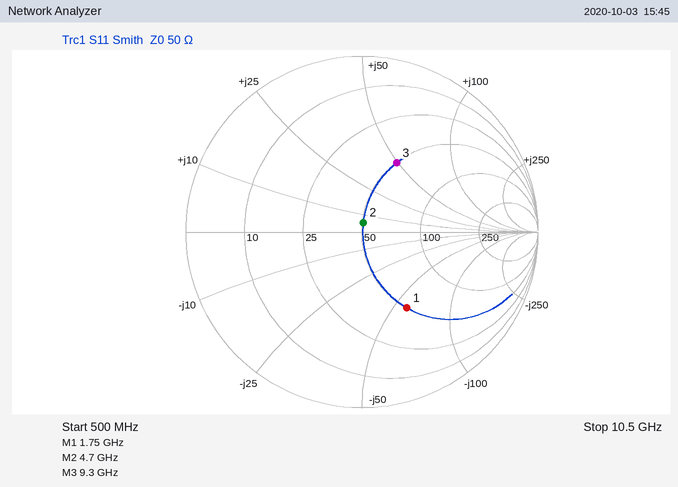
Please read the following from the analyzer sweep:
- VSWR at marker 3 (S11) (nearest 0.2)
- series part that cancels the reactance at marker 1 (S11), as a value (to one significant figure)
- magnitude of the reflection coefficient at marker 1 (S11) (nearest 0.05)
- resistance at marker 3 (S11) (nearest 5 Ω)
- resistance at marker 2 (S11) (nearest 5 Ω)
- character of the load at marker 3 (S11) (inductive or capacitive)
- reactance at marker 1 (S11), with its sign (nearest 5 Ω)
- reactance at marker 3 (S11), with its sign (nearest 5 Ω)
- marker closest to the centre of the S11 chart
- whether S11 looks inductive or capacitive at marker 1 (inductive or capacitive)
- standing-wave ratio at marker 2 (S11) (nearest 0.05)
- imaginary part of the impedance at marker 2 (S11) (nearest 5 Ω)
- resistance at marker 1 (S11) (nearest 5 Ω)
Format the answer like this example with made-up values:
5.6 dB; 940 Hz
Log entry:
2.6; 5 nH; 0.50; 50 Ω; 50 Ω; inductive; -60 Ω; +50 Ω; marker 2; capacitive; 1.10; +5 Ω; 50 Ω
